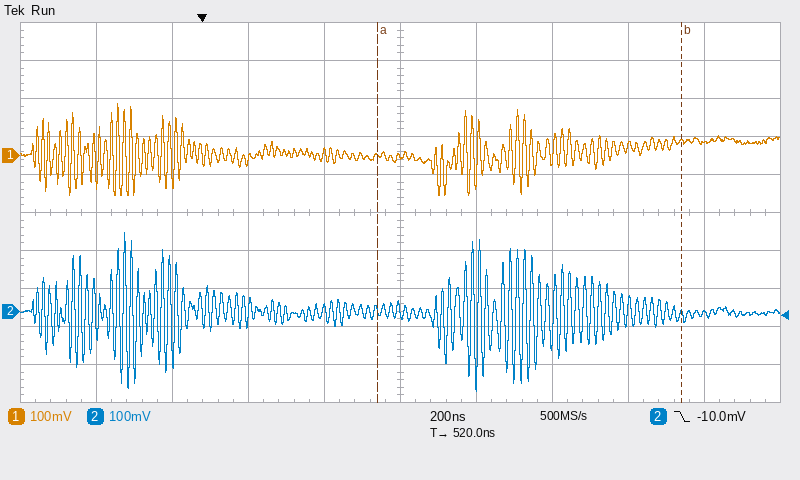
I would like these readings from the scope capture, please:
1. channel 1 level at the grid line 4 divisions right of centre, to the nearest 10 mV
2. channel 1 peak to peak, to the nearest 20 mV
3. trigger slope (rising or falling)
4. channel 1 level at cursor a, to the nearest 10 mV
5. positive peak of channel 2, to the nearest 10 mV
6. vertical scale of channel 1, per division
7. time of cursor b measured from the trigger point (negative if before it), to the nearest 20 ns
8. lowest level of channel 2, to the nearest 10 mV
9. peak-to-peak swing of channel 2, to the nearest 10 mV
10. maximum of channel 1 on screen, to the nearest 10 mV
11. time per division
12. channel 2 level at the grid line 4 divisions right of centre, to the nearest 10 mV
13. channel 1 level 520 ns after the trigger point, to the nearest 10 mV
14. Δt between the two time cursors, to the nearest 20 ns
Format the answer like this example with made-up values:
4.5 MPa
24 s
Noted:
30 mV
240 mV
falling
0 mV
210 mV
100 mV
+1.26 µs
-210 mV
420 mV
140 mV
200 ns
-10 mV
0 mV
800 ns
